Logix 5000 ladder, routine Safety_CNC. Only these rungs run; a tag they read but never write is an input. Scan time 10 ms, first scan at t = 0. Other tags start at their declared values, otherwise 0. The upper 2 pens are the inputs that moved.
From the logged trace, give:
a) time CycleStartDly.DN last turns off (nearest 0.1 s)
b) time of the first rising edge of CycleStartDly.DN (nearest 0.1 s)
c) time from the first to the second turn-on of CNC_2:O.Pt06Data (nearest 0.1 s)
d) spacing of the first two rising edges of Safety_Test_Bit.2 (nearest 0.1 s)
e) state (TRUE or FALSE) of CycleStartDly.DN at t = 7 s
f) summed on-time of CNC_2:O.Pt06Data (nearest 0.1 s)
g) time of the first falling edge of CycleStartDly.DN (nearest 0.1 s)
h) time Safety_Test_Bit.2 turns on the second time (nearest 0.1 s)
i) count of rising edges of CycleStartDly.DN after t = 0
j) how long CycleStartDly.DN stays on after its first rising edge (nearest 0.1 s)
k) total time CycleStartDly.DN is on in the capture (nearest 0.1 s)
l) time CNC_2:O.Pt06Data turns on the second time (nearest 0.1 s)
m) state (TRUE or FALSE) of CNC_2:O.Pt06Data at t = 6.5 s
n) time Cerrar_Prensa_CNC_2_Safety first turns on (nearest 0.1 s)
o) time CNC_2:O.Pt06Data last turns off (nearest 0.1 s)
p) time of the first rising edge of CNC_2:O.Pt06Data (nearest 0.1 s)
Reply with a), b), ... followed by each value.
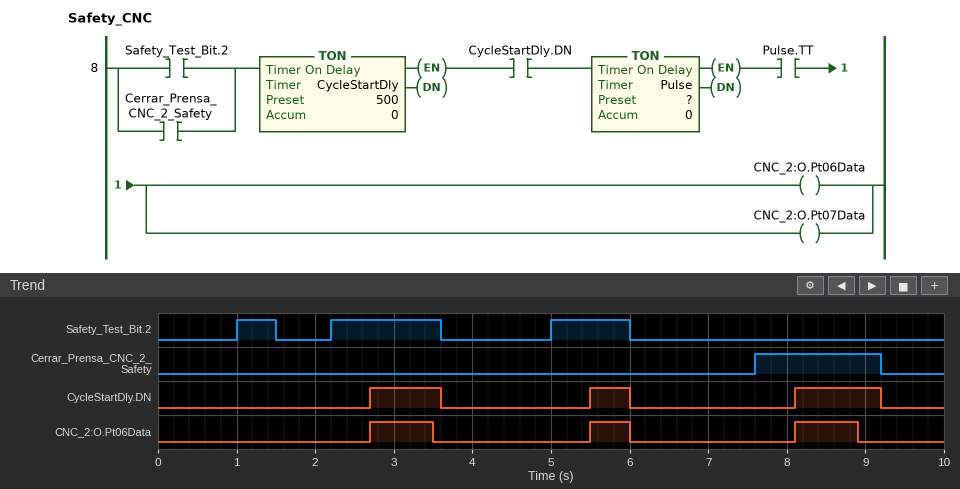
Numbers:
a) 9.2 s
b) 2.7 s
c) 2.8 s
d) 1.2 s
e) FALSE
f) 2.1 s
g) 3.6 s
h) 2.2 s
i) 3
j) 0.9 s
k) 2.5 s
l) 5.5 s
m) FALSE
n) 7.6 s
o) 8.9 s
p) 2.7 s
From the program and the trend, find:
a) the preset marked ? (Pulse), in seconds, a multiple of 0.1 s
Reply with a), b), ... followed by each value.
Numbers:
a) 0.8 s
